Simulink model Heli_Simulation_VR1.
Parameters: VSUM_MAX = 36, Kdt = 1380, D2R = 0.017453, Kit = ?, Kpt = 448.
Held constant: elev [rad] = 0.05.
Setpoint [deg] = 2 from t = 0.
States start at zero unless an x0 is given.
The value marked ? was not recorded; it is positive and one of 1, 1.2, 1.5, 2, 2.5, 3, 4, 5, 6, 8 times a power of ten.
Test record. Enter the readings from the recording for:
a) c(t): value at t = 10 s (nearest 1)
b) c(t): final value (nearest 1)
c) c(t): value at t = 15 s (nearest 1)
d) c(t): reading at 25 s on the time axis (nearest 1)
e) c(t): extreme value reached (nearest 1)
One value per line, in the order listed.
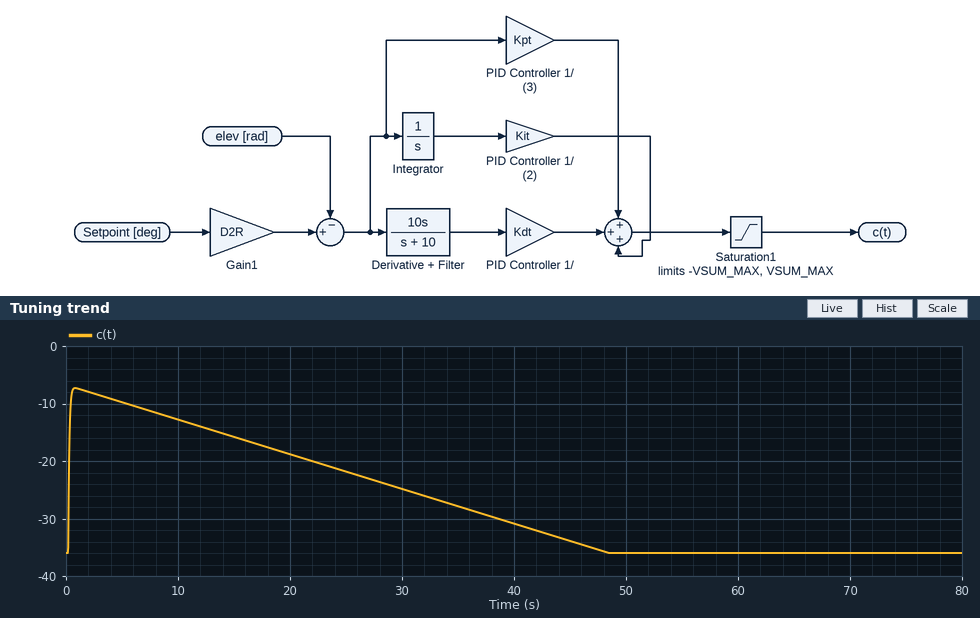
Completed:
-13
-36
-16
-22
-7
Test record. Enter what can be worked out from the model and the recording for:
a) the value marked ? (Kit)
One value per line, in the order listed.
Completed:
40
